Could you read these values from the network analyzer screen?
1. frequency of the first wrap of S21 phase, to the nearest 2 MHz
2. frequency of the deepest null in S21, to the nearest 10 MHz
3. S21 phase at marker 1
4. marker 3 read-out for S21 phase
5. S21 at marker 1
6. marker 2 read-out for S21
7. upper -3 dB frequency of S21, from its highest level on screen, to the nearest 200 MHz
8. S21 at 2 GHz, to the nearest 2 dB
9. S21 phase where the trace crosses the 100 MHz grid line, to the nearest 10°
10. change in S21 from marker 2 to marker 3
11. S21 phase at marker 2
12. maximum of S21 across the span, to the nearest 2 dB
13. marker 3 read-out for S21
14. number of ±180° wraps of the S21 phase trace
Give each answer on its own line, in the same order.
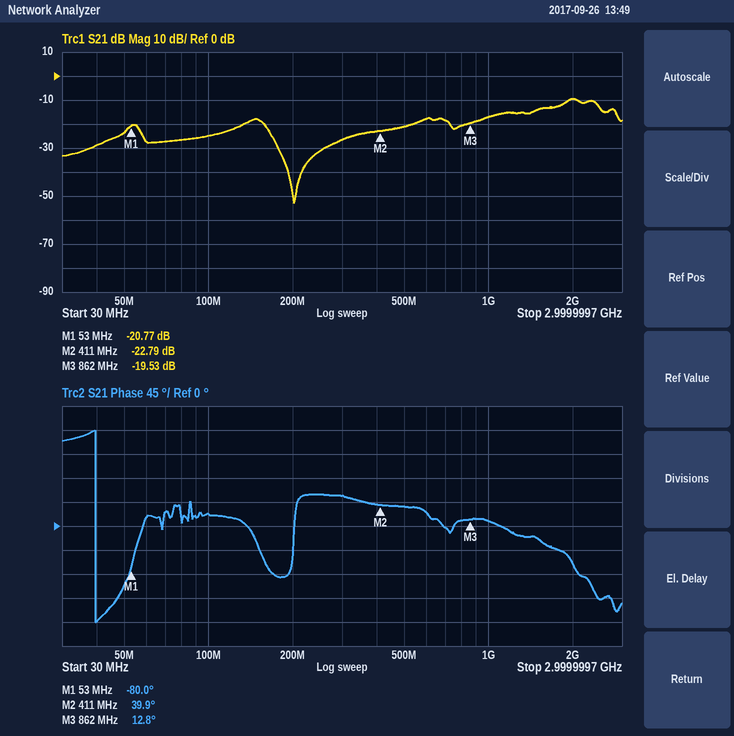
40 MHz
200 MHz
-80.0°
12.8°
-20.77 dB
-22.79 dB
2.4 GHz
-10 dB
20°
3.26 dB
39.9°
-10 dB
-19.53 dB
1
